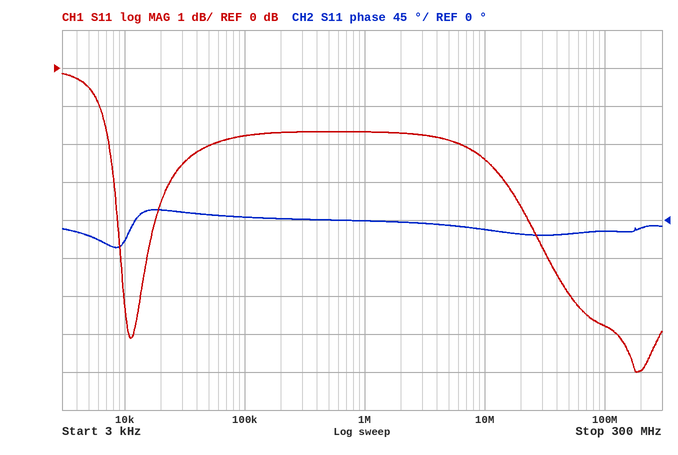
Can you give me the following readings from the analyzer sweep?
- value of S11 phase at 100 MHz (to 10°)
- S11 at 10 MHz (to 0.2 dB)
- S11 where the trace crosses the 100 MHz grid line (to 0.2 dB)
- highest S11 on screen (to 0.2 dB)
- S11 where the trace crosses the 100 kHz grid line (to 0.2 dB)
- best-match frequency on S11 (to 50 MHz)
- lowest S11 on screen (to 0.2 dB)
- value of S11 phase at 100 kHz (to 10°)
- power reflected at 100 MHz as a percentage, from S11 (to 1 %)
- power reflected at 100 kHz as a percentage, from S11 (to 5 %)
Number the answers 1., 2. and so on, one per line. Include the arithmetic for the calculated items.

1. -10°
2. -2.4 dB
3. -6.8 dB
4. -0.2 dB
5. -1.8 dB
6. 200 MHz
7. -8.0 dB
8. 0°
9. 10^(-6.8/10) ≈ 21 %
10. 10^(-1.8/10) ≈ 66.1 %, so 65 % to the nearest 5 %
